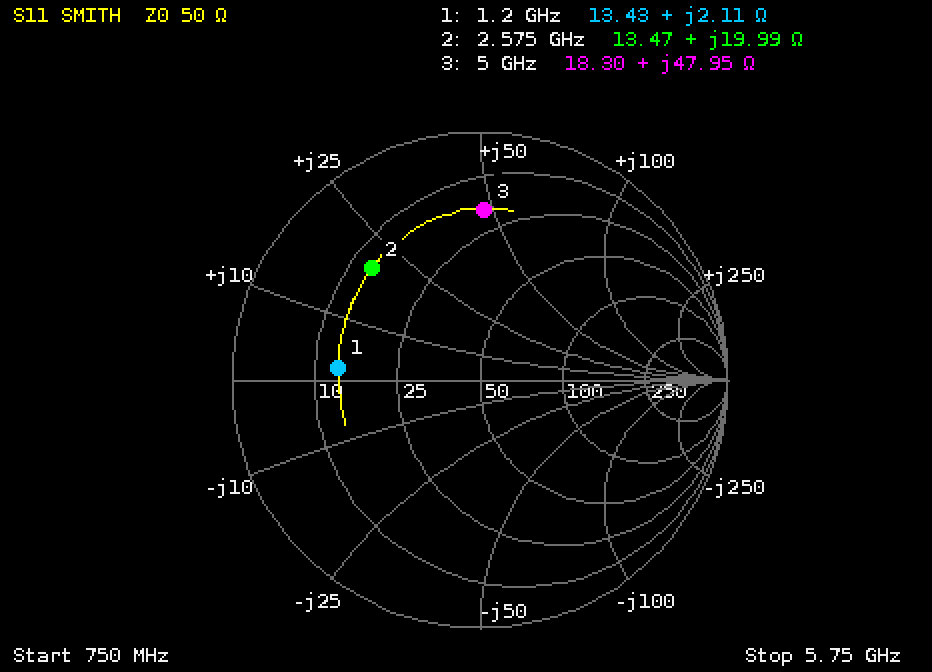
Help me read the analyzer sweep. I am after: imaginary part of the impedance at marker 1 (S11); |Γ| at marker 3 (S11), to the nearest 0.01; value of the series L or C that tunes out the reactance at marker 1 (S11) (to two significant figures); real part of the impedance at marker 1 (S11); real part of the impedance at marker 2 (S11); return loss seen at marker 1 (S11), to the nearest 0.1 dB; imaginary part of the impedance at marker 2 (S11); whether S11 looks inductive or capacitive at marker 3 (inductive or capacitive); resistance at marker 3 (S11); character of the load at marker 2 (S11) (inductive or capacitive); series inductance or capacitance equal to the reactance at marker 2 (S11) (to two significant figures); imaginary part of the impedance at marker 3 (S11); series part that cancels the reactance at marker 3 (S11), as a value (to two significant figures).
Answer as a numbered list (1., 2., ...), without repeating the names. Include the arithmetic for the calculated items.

1. +2.11 Ω
2. 0.69
3. C = 1/(2π × 1.2 GHz × 2.11 Ω) ≈ 63 pF
4. 13.43 Ω
5. 13.47 Ω
6. 4.8 dB
7. +19.99 Ω
8. inductive
9. 18.30 Ω
10. inductive
11. L = 19.99 Ω/(2π × 2.575 GHz) ≈ 1.2 nH
12. +47.95 Ω
13. C = 1/(2π × 5 GHz × 47.95 Ω) ≈ 664 fF, so 660 fF to two significant figures
